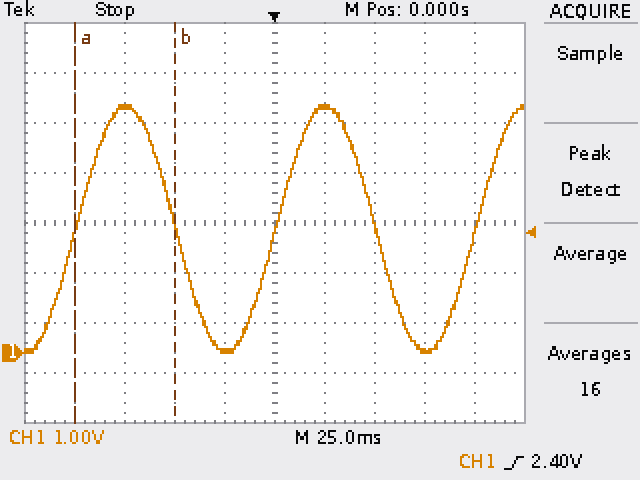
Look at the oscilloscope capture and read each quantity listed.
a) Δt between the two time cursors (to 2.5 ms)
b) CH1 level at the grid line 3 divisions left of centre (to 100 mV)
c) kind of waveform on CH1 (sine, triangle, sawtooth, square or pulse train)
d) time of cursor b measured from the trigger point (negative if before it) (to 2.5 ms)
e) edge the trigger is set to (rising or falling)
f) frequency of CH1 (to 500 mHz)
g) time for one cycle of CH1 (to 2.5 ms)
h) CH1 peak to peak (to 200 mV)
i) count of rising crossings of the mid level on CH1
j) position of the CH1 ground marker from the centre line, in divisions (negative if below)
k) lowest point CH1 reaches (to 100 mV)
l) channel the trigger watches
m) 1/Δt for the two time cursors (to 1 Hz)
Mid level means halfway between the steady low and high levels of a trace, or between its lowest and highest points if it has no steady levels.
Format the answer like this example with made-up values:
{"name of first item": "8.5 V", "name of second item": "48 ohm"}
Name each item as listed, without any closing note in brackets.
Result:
{"Δt between the two time cursors": "50.0 ms", "CH1 level at the grid line 3 divisions left of centre": "4.9 V", "kind of waveform on CH1": "sine", "time of cursor b measured from the trigger point (negative if before it)": "-50.0 ms", "edge the trigger is set to": "rising", "frequency of CH1": "10.0 Hz", "time for one cycle of CH1": "100.0 ms", "CH1 peak to peak": "5.0 V", "count of rising crossings of the mid level on CH1": "3", "position of the CH1 ground marker from the centre line, in divisions": "-2.6 div", "lowest point CH1 reaches": "0.0 V", "channel the trigger watches": "CH1", "1/Δt for the two time cursors": "20 Hz"}
